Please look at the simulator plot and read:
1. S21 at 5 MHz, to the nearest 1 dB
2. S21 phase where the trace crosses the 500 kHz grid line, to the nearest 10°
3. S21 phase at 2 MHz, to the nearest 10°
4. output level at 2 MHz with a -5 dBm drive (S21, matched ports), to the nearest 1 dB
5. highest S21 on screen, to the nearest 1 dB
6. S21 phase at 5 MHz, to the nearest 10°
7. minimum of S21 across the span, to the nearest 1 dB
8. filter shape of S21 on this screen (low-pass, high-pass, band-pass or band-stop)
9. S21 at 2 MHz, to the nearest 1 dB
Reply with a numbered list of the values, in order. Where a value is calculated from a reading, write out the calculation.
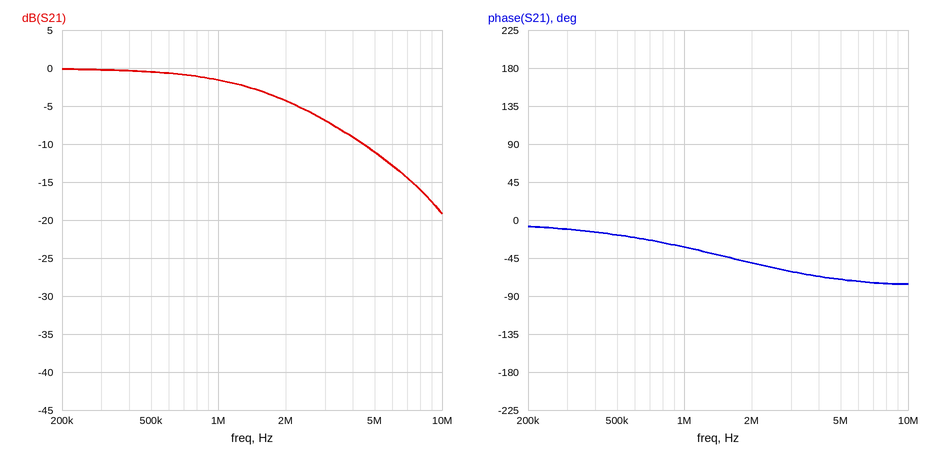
1. -11 dB
2. -20°
3. -50°
4. -5 dBm + (-4 dB) = -9 dBm
5. 0 dB
6. -70°
7. -19 dB
8. low-pass
9. -4 dB
